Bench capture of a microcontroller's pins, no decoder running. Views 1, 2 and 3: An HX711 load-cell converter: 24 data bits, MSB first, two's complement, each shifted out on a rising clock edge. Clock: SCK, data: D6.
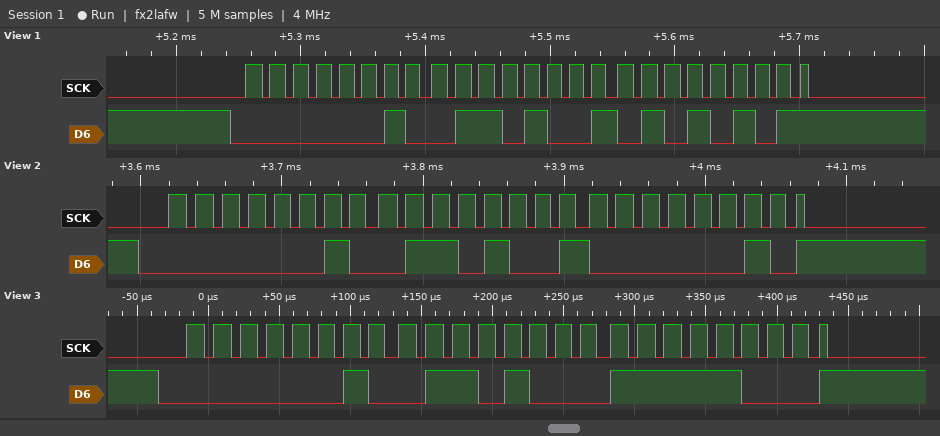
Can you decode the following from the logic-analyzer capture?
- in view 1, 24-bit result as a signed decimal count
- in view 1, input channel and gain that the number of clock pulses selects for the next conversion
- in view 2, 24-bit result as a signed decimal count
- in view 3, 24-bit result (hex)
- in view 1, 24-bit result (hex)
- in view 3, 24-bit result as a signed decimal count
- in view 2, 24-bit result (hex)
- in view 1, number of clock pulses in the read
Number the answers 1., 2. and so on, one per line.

1. 158037
2. channel A, gain 128
3. 157954
4. 0x0268F8
5. 0x026955
6. 157944
7. 0x026902
8. 25
